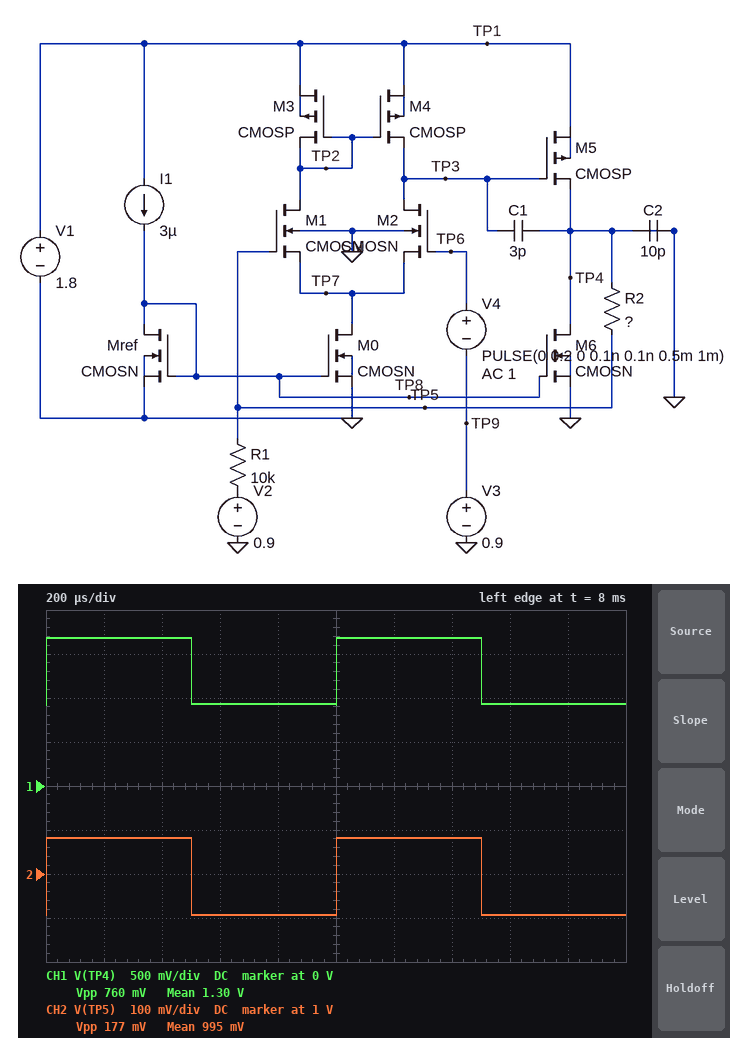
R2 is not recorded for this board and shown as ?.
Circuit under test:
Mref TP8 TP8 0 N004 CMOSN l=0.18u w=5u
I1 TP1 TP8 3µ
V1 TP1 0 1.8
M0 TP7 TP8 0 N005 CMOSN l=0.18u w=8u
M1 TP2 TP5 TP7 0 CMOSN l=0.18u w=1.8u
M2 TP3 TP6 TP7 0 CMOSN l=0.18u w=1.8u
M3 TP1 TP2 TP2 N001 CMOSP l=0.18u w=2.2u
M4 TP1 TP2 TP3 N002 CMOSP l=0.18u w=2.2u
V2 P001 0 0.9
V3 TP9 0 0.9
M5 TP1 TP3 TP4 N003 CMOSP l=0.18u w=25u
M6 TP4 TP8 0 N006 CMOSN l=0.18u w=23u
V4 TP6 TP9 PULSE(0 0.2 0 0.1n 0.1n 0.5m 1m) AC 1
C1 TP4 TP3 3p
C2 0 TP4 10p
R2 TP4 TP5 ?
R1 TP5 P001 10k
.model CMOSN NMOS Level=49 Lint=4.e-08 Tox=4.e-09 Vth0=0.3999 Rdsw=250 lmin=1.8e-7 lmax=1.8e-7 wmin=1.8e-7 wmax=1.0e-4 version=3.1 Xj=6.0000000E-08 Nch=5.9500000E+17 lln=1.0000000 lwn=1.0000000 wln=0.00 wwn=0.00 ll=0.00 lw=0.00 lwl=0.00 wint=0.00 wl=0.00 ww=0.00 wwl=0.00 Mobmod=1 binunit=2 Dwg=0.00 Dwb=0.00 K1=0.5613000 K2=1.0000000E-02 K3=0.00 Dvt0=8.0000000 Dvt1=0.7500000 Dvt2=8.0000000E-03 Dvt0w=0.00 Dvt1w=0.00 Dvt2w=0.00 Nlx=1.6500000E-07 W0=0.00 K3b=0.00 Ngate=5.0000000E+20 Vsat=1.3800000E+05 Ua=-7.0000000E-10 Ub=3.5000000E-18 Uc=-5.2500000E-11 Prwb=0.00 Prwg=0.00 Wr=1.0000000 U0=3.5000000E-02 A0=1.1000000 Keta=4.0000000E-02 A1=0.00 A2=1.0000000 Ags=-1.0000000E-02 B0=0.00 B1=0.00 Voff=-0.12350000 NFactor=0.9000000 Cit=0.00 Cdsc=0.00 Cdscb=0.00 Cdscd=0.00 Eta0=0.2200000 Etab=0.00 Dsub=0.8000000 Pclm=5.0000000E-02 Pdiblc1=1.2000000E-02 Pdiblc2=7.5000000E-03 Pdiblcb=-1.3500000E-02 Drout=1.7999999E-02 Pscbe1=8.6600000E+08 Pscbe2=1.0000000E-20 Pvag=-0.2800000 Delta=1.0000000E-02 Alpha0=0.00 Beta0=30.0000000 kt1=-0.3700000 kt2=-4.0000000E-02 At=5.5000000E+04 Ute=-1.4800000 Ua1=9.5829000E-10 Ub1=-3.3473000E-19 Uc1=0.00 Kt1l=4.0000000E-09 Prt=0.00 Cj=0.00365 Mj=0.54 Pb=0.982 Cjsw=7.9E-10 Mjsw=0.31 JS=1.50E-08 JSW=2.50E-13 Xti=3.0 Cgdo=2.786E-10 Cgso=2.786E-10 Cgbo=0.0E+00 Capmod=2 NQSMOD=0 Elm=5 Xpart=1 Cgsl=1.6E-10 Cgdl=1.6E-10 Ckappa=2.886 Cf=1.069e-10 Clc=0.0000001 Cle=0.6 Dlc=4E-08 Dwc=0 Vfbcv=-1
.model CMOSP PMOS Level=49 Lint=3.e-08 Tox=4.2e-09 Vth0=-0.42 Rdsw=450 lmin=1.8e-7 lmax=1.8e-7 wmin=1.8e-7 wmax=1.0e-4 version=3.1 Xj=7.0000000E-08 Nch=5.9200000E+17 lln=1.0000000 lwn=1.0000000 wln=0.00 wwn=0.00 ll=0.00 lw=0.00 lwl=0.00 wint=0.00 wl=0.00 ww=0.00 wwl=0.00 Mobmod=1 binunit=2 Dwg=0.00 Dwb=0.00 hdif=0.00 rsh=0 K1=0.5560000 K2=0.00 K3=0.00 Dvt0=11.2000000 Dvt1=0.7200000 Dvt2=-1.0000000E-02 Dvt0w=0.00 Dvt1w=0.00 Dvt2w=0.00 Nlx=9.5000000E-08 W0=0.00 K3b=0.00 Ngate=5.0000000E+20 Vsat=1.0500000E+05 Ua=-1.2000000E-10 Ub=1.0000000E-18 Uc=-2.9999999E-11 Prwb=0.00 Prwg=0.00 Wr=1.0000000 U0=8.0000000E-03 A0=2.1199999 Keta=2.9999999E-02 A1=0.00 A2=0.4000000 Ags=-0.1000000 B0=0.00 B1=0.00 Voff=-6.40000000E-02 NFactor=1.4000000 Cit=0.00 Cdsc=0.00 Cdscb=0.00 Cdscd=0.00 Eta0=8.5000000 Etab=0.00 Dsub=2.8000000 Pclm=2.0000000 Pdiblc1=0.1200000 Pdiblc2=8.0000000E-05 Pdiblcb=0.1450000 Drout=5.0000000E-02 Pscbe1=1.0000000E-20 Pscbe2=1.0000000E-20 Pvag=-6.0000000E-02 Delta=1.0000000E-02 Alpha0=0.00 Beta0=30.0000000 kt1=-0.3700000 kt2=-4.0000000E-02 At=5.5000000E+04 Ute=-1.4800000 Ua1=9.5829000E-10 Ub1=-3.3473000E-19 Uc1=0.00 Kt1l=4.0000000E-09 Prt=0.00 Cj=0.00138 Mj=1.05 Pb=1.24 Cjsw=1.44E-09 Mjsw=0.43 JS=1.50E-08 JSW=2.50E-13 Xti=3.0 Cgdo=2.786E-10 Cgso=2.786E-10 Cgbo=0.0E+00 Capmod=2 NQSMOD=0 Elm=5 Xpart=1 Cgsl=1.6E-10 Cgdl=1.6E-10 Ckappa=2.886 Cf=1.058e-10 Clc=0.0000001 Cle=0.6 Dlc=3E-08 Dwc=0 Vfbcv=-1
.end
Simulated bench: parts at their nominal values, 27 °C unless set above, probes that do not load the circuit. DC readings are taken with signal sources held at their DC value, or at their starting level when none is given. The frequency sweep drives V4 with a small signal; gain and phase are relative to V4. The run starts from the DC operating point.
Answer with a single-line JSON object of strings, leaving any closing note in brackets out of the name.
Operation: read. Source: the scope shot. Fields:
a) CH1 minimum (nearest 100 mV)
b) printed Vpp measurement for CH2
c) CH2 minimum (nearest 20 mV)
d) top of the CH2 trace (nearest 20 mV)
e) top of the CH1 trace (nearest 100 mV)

{"CH1 minimum": "900 mV", "printed Vpp measurement for CH2": "177 mV", "CH2 minimum": "900 mV", "top of the CH2 trace": "1.08 V", "top of the CH1 trace": "1.7 V"}
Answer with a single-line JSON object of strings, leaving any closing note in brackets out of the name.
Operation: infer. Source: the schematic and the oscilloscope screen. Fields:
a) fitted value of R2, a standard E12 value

{"fitted value of R2, a standard E12 value": "33 kΩ"}
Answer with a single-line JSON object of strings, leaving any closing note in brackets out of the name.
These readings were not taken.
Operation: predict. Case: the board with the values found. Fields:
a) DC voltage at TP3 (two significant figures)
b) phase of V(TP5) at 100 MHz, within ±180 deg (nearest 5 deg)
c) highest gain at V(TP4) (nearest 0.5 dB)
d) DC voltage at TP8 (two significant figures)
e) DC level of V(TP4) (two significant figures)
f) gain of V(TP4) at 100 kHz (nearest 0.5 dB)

{"DC voltage at TP3": "1.5 V", "phase of V(TP5) at 100 MHz, within ±180 deg": "110 deg", "highest gain at V(TP4)": "12.0 dB", "DC voltage at TP8": "310 mV", "DC level of V(TP4)": "910 mV", "gain of V(TP4) at 100 kHz": "11.5 dB"}
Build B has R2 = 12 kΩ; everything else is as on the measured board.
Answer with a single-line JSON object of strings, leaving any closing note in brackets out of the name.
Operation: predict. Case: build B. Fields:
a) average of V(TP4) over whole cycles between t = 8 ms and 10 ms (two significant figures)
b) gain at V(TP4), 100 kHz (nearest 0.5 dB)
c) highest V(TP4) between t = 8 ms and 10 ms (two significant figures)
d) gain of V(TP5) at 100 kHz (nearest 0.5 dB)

{"average of V(TP4) over whole cycles between t = 8 ms and 10 ms": "1.1 V", "gain at V(TP4), 100 kHz": "6.5 dB", "highest V(TP4) between t = 8 ms and 10 ms": "1.3 V", "gain of V(TP5) at 100 kHz": "-0.5 dB"}
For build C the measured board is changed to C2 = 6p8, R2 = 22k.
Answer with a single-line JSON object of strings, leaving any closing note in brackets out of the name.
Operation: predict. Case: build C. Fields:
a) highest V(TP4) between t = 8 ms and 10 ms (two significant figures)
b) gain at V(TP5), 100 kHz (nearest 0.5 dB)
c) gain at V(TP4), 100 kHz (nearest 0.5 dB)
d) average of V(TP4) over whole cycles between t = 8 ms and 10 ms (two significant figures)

{"highest V(TP4) between t = 8 ms and 10 ms": "1.5 V", "gain at V(TP5), 100 kHz": "-0.5 dB", "gain at V(TP4), 100 kHz": "9.5 dB", "average of V(TP4) over whole cycles between t = 8 ms and 10 ms": "1.2 V"}
